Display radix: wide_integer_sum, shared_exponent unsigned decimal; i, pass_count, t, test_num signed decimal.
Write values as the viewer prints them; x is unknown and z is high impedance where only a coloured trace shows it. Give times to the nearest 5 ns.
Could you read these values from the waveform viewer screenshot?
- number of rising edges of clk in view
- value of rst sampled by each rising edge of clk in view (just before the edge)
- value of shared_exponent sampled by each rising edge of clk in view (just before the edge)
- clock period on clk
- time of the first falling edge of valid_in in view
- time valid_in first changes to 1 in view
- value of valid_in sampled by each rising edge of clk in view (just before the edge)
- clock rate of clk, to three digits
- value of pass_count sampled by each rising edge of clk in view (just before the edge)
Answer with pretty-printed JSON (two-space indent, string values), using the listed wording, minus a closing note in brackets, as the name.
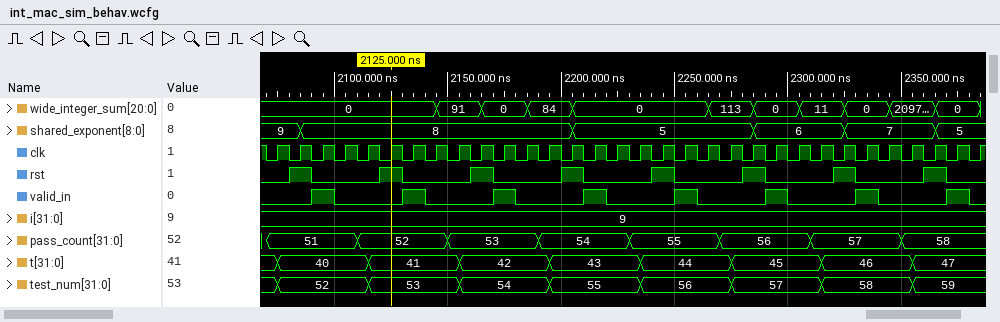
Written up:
{
  "number of rising edges of clk in view": "32",
  "value of rst sampled by each rising edge of clk in view": "0 1 0 0 0 1 0 0 0 1 0 0 0 1 0 0 0 1 0 0 0 1 0 0 0 1 0 0 0 1 0 0",
  "value of shared_exponent sampled by each rising edge of clk in view": "9, 9, 8, 8, 8, 8, 8, 8, 8, 8, 8, 8, 8, 8, 5, 5, 5, 5, 5, 5, 5, 5, 6, 6, 6, 6, 7, 7, 7, 7, 5, 5",
  "clock period on clk": "10 ns",
  "time of the first falling edge of valid_in in view": "2100 ns",
  "time valid_in first changes to 1 in view": "2090 ns",
  "value of valid_in sampled by each rising edge of clk in view": "0 0 1 0 0 0 1 0 0 0 1 0 0 0 1 0 0 0 1 0 0 0 1 0 0 0 1 0 0 0 1 0",
  "clock rate of clk, to three digits": "100 MHz",
  "value of pass_count sampled by each rising edge of clk in view": "51, 51, 51, 51, 52, 52, 52, 52, 53, 53, 53, 53, 54, 54, 54, 54, 55, 55, 55, 55, 56, 56, 56, 56, 57, 57, 57, 57, 58, 58, 58, 58"
}
